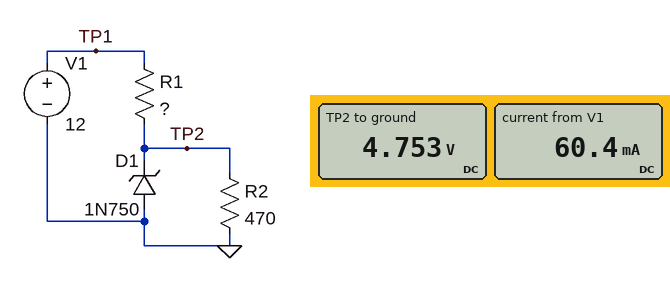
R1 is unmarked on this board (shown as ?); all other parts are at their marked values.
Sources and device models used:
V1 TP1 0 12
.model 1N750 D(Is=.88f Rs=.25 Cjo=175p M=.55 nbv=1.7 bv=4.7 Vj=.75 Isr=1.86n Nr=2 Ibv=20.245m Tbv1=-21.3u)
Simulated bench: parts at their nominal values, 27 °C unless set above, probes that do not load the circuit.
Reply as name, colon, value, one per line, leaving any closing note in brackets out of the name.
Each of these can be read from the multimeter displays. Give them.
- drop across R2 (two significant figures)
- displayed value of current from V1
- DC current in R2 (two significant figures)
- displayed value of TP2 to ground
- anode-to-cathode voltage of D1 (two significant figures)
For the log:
drop across R2: 4.8 V
displayed value of current from V1: 60.4 mA
DC current in R2: 10 mA
displayed value of TP2 to ground: 4.753 V
anode-to-cathode voltage of D1: -4.8 V
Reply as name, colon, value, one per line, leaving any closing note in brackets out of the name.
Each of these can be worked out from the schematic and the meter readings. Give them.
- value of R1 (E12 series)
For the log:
value of R1: 120 Ω
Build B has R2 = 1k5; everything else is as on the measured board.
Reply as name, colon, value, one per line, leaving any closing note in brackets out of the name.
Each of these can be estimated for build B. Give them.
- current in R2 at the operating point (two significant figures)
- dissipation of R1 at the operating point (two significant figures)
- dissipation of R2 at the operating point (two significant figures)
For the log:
current in R2 at the operating point: 3.2 mA
dissipation of R1 at the operating point: 440 mW
dissipation of R2 at the operating point: 15 mW
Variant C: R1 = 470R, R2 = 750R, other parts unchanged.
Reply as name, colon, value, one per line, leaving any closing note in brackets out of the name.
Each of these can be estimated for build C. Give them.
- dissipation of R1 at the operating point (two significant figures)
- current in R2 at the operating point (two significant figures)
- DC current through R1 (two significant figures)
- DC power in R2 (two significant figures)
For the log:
dissipation of R1 at the operating point: 110 mW
current in R2 at the operating point: 6.2 mA
DC current through R1: 16 mA
DC power in R2: 29 mW
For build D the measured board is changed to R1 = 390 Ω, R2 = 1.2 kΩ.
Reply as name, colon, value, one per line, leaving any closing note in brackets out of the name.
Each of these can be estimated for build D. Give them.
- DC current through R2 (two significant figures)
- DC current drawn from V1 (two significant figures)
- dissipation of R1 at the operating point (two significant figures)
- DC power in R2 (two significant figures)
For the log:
DC current through R2: 3.9 mA
DC current drawn from V1: 19 mA
dissipation of R1 at the operating point: 140 mW
DC power in R2: 18 mW
